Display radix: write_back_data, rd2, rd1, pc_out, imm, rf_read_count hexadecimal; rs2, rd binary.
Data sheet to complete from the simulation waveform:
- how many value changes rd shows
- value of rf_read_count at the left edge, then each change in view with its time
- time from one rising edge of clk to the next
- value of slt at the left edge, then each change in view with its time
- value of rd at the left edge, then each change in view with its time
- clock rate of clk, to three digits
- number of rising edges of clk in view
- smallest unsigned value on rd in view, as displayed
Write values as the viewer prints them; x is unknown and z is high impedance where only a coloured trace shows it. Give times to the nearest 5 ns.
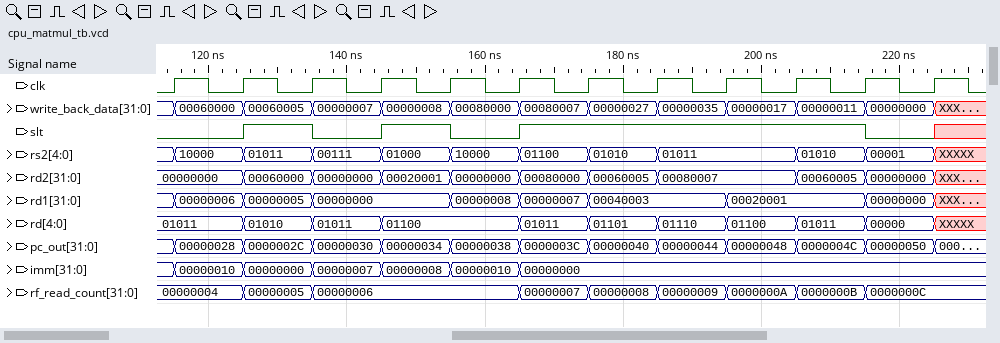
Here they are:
10
00000004, 00000005 at 125 ns, 00000006 at 135 ns, 00000007 at 165 ns, 00000008 at 175 ns, 00000009 at 185 ns, 0000000A at 195 ns, 0000000B at 205 ns, 0000000C at 215 ns
10 ns
0, 1 at 125 ns, 0 at 135 ns, 1 at 145 ns, 0 at 155 ns, 1 at 165 ns, 0 at 215 ns, x at 225 ns
01011, 01010 at 125 ns, 01011 at 135 ns, 01100 at 145 ns, 01011 at 165 ns, 01101 at 175 ns, 01110 at 185 ns, 01100 at 195 ns, 01011 at 205 ns, 00000 at 215 ns, XXXXX at 225 ns
100 MHz
12
00000
